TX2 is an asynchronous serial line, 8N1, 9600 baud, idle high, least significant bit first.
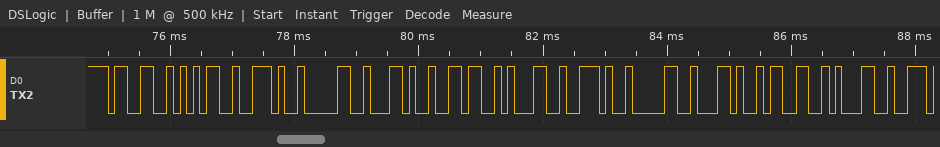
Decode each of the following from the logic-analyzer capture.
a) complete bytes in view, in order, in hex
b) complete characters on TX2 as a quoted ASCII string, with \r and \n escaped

0x33 0x35 0x2E 0x30 0x2C 0x36 0x31 0x2E 0x30 0x2C 0x33 0x31
"35.0,61.0,31"
